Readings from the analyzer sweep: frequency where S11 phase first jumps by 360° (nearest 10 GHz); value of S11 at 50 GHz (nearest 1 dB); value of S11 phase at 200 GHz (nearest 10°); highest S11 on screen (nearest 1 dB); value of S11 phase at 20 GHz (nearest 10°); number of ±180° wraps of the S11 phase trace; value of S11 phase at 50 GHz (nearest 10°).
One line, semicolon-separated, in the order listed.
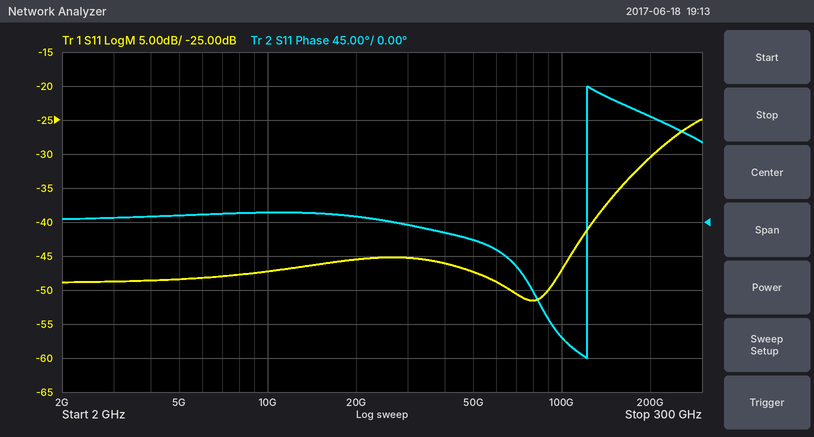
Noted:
120 GHz; -47 dB; 140°; -25 dB; 10°; 1; -20°
